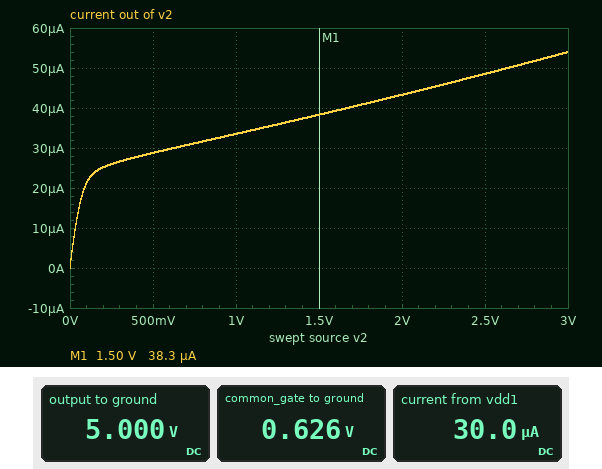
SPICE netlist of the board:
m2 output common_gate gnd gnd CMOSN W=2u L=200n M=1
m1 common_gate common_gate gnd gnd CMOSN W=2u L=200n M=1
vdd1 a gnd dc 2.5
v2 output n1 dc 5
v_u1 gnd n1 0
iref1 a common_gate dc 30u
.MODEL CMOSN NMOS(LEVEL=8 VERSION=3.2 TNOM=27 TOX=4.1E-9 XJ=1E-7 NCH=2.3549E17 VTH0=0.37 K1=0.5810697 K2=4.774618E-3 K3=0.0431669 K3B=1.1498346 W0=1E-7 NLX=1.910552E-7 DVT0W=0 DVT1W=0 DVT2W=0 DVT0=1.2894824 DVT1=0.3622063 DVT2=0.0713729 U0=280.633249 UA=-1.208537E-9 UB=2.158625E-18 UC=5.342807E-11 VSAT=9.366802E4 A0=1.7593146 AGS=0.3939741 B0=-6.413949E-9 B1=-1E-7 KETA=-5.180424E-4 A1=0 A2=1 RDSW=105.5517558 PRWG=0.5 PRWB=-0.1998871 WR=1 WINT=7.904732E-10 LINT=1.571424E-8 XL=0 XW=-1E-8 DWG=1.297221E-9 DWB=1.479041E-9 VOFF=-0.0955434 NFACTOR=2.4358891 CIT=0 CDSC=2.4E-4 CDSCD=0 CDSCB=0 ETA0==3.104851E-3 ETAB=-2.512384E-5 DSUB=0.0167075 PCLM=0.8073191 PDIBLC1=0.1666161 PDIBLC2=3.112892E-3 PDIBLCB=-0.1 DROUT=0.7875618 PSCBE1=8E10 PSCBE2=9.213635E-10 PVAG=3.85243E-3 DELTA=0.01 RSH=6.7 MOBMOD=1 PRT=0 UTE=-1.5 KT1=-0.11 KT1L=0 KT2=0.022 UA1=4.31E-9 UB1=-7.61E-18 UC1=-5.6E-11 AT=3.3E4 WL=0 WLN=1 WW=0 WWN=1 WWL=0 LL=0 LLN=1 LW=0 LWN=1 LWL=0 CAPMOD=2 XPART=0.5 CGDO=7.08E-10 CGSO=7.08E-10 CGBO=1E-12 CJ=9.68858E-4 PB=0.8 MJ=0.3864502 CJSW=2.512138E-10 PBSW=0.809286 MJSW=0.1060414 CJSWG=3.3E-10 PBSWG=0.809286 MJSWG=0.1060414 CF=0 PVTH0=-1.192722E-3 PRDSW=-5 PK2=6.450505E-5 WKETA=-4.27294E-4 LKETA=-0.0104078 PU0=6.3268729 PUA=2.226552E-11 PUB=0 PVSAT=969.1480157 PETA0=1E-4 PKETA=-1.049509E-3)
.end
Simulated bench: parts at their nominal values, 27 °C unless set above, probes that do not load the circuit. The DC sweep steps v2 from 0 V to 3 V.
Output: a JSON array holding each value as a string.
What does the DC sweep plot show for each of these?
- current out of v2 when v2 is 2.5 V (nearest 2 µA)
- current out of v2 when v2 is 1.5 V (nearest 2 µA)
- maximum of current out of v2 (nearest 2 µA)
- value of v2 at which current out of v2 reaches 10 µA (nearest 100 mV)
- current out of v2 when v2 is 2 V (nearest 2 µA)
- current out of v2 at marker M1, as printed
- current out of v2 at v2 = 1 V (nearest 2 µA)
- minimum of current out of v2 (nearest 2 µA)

["48 µA", "38 µA", "54 µA", "0 V", "44 µA", "38.3 µA", "34 µA", "0 A"]
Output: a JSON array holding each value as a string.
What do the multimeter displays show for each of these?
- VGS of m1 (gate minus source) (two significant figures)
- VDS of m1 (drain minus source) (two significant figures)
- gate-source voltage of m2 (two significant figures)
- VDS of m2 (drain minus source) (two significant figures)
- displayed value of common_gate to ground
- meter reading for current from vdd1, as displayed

["630 mV", "630 mV", "630 mV", "5.0 V", "0.626 V", "30.0 µA"]
